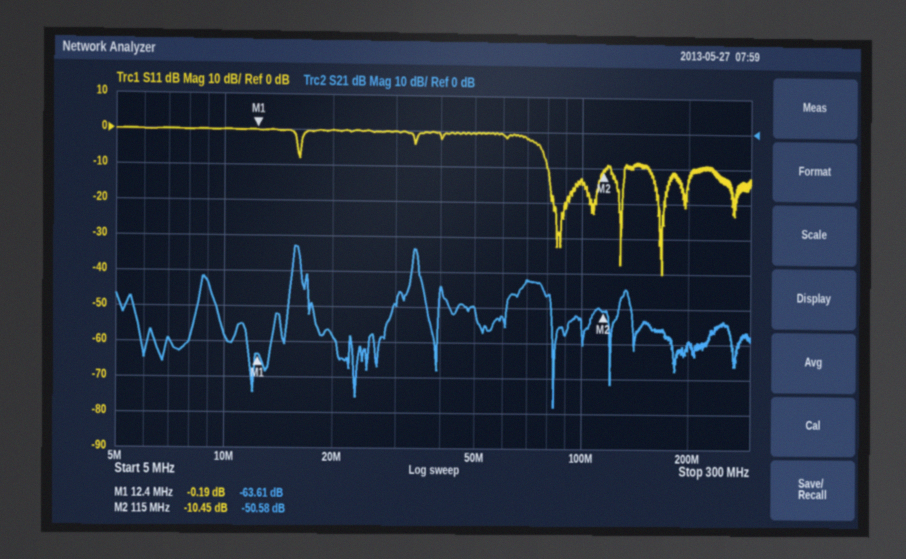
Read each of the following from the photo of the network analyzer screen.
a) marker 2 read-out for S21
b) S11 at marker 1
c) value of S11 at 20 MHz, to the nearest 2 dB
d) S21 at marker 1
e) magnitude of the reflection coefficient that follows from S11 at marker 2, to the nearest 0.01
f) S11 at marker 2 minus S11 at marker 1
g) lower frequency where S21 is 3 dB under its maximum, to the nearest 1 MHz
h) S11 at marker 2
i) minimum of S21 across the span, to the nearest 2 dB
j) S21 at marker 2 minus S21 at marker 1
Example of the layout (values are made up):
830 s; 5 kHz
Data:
-50.58 dB; -0.19 dB; 0 dB; -63.61 dB; 0.30; -10.26 dB; 16 MHz; -10.45 dB; -78 dB; 13.03 dB
